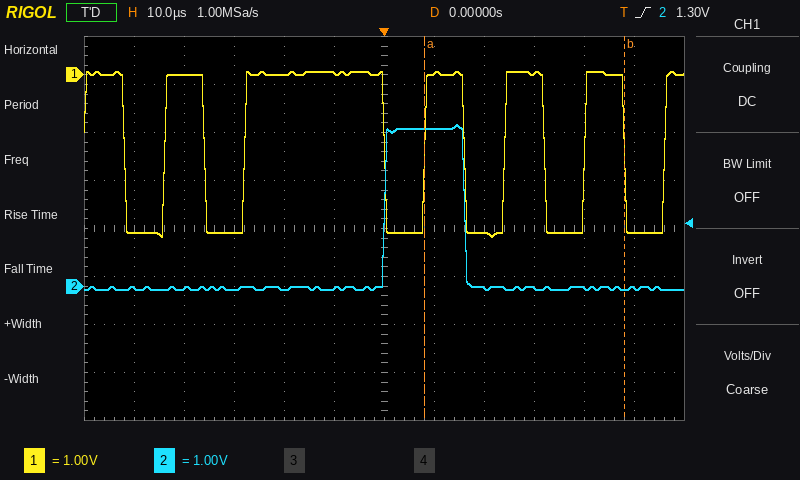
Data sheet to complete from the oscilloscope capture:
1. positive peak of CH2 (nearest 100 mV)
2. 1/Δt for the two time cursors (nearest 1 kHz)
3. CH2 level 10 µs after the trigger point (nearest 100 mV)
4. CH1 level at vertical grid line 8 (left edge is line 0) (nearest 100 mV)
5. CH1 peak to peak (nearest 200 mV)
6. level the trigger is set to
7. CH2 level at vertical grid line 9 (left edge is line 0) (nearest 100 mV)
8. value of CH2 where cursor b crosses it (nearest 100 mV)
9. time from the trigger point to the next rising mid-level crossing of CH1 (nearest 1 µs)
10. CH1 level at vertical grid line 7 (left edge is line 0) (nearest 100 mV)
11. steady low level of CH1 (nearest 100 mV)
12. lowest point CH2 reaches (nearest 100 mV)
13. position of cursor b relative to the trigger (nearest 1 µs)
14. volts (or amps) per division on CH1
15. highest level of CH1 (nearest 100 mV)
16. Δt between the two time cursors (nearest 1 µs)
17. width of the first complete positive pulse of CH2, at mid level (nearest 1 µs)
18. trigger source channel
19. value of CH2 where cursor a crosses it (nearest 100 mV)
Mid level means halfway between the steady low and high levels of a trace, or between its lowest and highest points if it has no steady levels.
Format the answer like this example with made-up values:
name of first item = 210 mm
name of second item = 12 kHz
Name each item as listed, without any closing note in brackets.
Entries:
positive peak of CH2 = 3.4 V
1/Δt for the two time cursors = 25 kHz
CH2 level 10 µs after the trigger point = 3.3 V
CH1 level at vertical grid line 8 (left edge is line 0) = -3.3 V
CH1 peak to peak = 3.4 V
level the trigger is set to = 1.30 V
CH2 level at vertical grid line 9 (left edge is line 0) = 0.0 V
value of CH2 where cursor b crosses it = -100 mV
time from the trigger point to the next rising mid-level crossing of CH1 = 8 µs
CH1 level at vertical grid line 7 (left edge is line 0) = 0.0 V
steady low level of CH1 = -3.3 V
lowest point CH2 reaches = -100 mV
position of cursor b relative to the trigger = +48 µs
volts (or amps) per division on CH1 = 1 V
highest level of CH1 = 100 mV
Δt between the two time cursors = 40 µs
width of the first complete positive pulse of CH2, at mid level = 16 µs
trigger source channel = CH2
value of CH2 where cursor a crosses it = 3.3 V
